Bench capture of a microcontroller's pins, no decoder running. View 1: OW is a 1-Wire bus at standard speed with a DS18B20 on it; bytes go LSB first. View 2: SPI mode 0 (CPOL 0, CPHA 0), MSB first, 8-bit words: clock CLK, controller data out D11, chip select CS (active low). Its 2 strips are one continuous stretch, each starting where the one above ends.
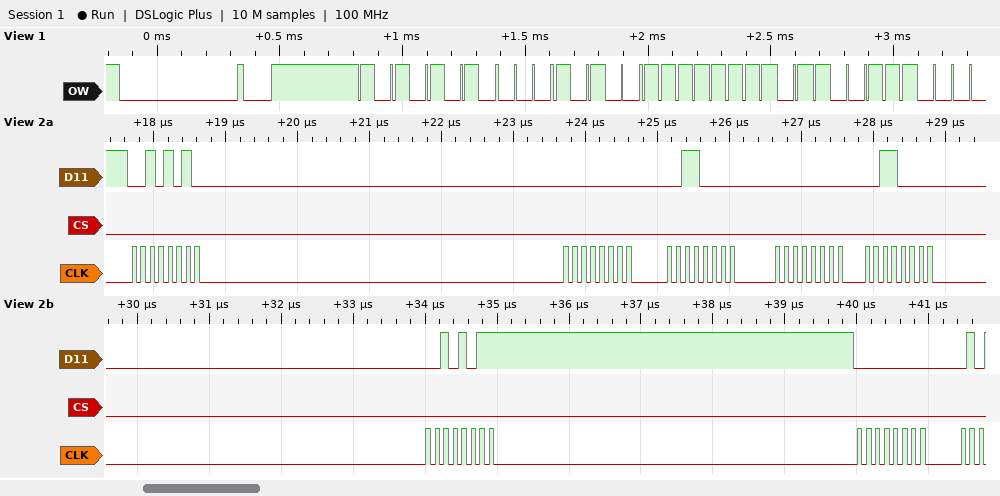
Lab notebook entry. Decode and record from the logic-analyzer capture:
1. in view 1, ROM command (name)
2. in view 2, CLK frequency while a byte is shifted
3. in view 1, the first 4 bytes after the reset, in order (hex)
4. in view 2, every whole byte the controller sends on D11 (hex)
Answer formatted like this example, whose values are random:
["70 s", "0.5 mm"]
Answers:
["Match ROM", "8 MHz", "55 28 FF E6", "0x2A 0x00 0x30 0x00 0x30 0x2B 0x00"]
